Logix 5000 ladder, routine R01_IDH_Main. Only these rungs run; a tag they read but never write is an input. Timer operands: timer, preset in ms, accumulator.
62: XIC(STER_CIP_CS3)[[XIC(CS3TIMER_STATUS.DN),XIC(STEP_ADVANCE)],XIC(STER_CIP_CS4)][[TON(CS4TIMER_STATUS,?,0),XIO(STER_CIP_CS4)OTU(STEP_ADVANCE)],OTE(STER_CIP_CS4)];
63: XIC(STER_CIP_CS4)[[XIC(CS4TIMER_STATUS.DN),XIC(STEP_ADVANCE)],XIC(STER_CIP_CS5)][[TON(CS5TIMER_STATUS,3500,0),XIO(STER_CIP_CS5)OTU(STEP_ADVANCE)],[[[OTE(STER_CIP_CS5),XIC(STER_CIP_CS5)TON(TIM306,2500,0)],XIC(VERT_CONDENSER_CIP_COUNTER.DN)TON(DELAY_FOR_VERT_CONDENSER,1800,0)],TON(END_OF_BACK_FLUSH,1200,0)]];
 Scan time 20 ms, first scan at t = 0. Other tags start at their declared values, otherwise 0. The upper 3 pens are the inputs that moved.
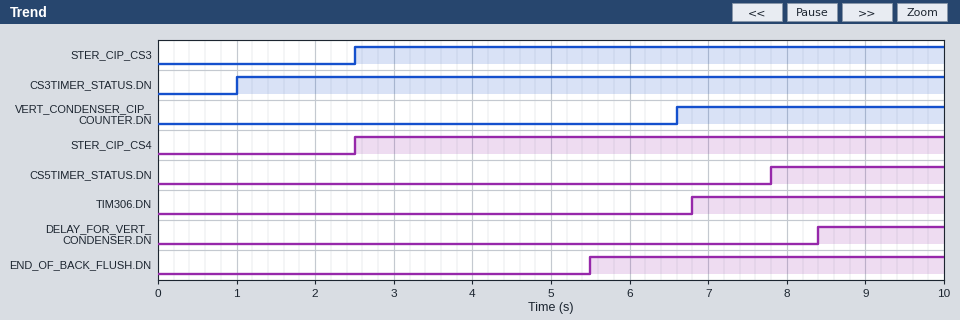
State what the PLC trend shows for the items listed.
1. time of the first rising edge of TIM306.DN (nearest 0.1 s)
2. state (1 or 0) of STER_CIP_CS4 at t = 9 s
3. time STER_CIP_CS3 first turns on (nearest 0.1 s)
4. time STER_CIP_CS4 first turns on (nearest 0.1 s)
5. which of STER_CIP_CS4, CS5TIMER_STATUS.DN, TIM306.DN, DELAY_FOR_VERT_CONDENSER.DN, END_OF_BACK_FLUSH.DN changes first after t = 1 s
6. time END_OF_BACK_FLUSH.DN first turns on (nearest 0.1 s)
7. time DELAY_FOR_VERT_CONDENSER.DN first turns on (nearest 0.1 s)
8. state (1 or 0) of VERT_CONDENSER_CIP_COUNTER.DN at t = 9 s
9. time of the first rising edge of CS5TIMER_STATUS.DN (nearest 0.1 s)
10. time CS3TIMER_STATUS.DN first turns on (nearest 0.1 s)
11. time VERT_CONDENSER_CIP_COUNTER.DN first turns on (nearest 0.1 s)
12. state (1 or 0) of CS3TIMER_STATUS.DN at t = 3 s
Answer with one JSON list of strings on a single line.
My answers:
["6.8 s", "1", "2.5 s", "2.5 s", "STER_CIP_CS4", "5.5 s", "8.4 s", "1", "7.8 s", "1.0 s", "6.6 s", "1"]
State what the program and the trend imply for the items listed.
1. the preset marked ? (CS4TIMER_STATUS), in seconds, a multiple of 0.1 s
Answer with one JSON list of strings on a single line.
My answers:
["1.8 s"]
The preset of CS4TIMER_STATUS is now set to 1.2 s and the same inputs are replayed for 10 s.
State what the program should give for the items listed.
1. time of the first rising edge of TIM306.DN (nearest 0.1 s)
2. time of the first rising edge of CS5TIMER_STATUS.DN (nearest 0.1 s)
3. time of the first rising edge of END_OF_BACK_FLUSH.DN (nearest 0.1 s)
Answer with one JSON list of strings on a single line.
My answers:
["6.2 s", "7.2 s", "4.9 s"]
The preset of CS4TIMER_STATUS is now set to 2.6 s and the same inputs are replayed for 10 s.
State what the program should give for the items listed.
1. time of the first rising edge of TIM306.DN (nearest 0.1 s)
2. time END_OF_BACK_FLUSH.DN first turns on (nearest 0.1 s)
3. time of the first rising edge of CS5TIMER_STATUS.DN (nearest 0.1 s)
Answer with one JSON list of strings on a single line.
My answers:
["7.6 s", "6.3 s", "8.6 s"]
